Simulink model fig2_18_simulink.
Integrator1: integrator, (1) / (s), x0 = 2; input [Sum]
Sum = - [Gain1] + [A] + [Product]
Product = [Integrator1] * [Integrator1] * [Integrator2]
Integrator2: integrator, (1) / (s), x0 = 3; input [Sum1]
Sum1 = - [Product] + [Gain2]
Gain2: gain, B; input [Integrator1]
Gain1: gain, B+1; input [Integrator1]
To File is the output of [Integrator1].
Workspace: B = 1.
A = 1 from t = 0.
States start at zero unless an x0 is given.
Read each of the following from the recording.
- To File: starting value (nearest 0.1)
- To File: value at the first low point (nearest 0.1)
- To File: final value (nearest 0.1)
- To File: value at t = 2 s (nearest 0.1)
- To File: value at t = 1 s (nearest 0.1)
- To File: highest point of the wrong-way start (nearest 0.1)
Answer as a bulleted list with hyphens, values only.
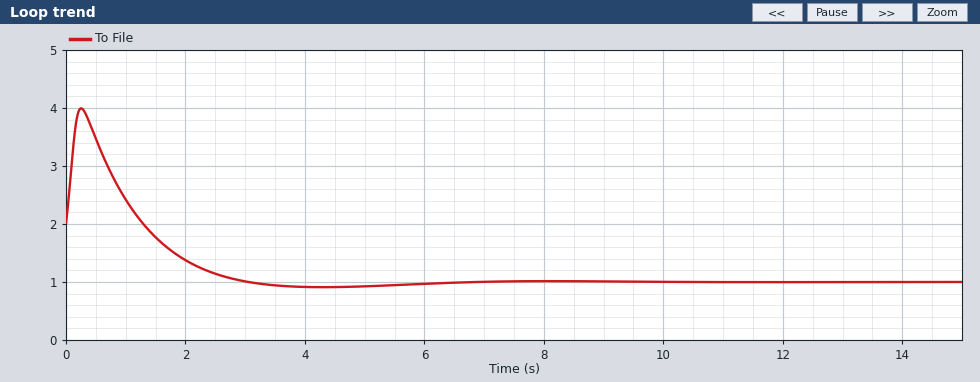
- 2.0
- 0.9
- 1.0
- 1.4
- 2.4
- 4.0
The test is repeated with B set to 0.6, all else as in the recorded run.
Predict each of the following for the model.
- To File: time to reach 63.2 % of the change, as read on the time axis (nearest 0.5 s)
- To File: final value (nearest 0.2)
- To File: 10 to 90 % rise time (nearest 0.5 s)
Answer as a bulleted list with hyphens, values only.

- 2.0 s
- 1.0
- 1.5 s
